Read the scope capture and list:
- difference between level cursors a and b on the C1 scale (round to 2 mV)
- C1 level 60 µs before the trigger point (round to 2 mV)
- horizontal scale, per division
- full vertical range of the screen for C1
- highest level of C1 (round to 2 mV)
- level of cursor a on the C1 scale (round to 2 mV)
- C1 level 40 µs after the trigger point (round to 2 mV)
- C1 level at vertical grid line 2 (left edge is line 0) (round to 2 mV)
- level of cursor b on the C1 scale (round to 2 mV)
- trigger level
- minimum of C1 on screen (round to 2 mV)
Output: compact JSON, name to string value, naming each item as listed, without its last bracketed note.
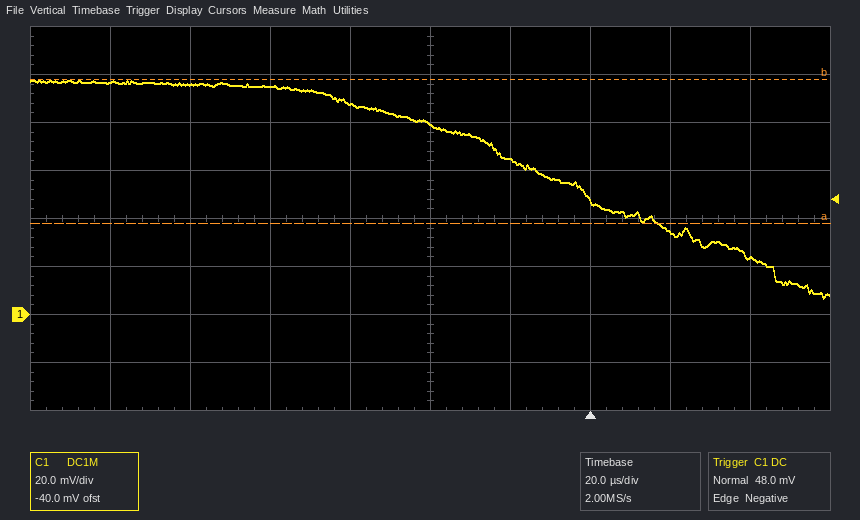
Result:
{"difference between level cursors a and b on the C1 scale": "60 mV", "C1 level 60 µs before the trigger point": "88 mV", "horizontal scale, per division": "20 µs", "full vertical range of the screen for C1": "160 mV", "highest level of C1": "98 mV", "level of cursor a on the C1 scale": "38 mV", "C1 level 40 µs after the trigger point": "24 mV", "C1 level at vertical grid line 2 (left edge is line 0)": "96 mV", "level of cursor b on the C1 scale": "98 mV", "trigger level": "48.0 mV", "minimum of C1 on screen": "6 mV"}
